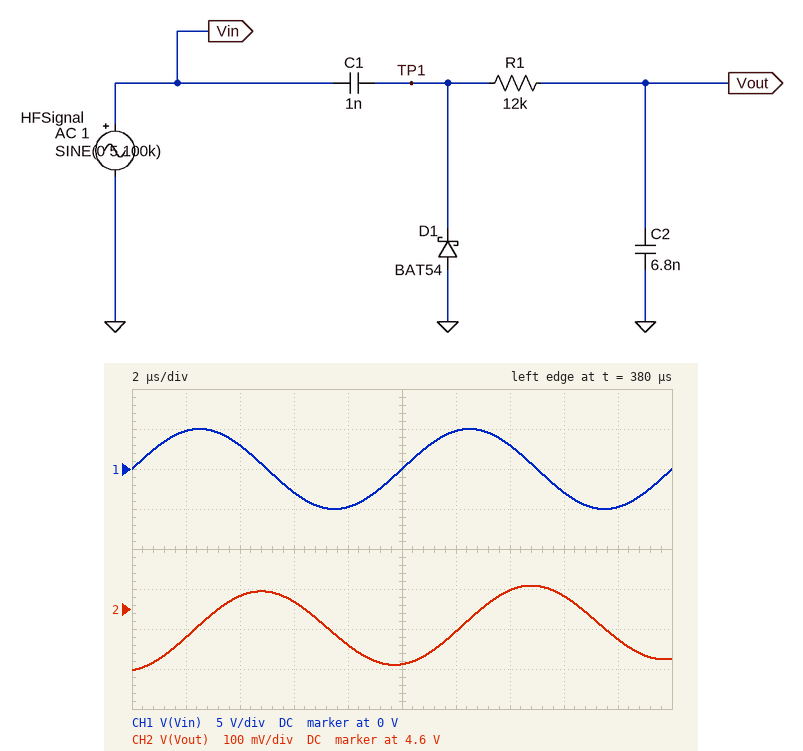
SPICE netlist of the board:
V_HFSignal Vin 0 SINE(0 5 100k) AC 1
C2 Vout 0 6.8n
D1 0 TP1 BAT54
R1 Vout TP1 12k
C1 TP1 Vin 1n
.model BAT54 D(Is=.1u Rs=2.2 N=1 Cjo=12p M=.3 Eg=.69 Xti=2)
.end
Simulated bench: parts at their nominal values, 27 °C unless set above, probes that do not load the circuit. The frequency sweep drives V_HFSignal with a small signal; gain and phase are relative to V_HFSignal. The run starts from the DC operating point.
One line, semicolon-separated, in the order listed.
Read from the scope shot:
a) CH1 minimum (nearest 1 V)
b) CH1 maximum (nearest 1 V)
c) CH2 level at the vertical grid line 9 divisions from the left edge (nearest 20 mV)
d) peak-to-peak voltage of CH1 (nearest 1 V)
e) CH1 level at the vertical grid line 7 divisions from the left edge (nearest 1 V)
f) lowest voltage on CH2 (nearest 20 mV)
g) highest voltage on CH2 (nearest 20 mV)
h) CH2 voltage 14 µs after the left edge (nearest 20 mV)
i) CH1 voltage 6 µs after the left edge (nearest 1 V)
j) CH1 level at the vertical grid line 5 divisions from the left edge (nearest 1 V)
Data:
-5 V; 5 V; 4.52 V; 10 V; 3 V; 4.44 V; 4.66 V; 4.64 V; -3 V; 0 V
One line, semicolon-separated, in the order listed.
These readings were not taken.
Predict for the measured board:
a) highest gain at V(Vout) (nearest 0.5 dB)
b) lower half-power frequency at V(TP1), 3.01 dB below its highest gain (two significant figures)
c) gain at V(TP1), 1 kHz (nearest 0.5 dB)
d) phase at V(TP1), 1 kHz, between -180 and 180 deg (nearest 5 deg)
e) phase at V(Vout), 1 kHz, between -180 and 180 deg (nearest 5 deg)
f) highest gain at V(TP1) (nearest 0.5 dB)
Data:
-18.0 dB; 15 kHz; -17.0 dB; 30 deg; 0 deg; 0 dB
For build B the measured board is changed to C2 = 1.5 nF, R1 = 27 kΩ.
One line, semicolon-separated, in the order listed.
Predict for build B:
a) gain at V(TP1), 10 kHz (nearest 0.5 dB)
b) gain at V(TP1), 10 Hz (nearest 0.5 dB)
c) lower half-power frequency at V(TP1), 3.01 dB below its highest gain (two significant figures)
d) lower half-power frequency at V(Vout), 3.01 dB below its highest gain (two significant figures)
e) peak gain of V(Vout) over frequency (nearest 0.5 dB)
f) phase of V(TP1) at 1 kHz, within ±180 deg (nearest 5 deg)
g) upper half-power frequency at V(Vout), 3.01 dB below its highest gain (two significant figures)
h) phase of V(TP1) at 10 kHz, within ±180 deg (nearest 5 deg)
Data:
-2.5 dB; -36.0 dB; 8.5 kHz; 230 Hz; -8.5 dB; 20 deg; 11 kHz; 25 deg
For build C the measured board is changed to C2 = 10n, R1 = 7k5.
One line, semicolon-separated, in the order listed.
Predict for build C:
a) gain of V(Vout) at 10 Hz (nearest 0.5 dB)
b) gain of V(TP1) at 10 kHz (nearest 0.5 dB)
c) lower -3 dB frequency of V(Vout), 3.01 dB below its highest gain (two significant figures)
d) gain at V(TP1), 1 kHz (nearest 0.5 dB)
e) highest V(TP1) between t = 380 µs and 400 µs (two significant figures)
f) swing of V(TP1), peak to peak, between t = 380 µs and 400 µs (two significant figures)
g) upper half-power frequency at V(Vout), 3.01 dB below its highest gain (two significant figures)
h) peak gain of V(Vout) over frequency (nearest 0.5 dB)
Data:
-36.0 dB; -8.0 dB; 54 Hz; -20.0 dB; 9.4 V; 9.6 V; 24 kHz; -21.0 dB
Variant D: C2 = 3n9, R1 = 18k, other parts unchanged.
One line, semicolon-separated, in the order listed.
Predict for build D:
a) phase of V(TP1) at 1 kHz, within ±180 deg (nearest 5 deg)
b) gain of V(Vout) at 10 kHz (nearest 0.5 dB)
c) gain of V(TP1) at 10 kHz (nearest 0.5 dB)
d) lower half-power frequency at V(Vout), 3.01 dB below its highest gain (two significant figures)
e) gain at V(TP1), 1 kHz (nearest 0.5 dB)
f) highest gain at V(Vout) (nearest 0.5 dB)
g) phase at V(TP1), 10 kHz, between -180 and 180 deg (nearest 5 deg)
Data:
25 deg; -16.5 dB; -3.5 dB; 120 Hz; -13.5 dB; -14.5 dB; 35 deg
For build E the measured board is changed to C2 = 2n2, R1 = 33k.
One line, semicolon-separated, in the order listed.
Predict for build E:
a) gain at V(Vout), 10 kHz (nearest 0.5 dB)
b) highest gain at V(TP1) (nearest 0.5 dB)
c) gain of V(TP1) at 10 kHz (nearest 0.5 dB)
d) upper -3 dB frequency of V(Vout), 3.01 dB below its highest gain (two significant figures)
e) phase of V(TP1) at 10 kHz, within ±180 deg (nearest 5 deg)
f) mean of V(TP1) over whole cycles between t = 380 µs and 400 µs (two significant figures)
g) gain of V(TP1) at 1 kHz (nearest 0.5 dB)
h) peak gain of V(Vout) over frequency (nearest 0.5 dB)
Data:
-15.0 dB; 0 dB; -2.0 dB; 7.7 kHz; 25 deg; 4.8 V; -10.0 dB; -11.0 dB
